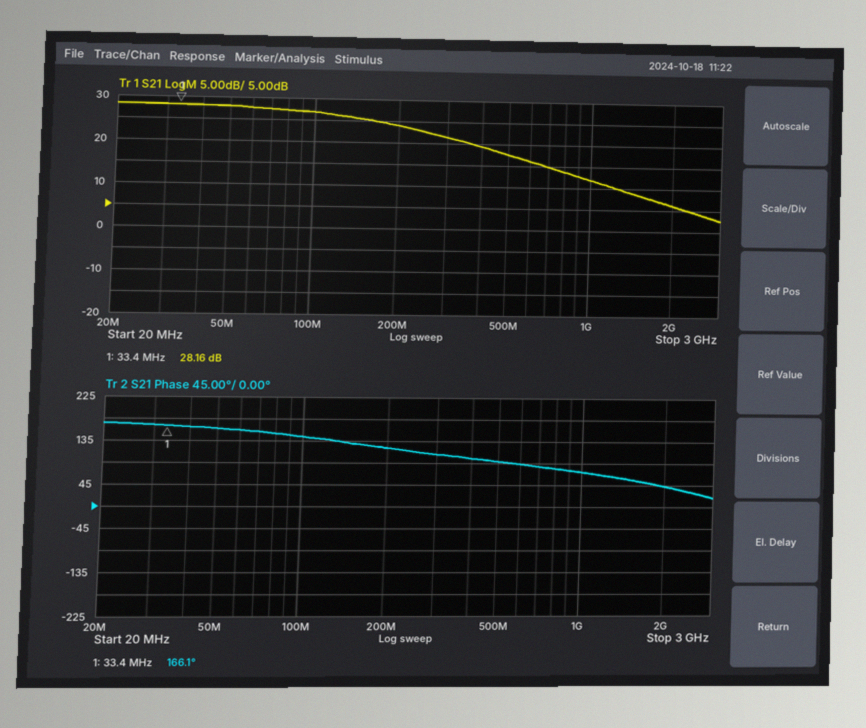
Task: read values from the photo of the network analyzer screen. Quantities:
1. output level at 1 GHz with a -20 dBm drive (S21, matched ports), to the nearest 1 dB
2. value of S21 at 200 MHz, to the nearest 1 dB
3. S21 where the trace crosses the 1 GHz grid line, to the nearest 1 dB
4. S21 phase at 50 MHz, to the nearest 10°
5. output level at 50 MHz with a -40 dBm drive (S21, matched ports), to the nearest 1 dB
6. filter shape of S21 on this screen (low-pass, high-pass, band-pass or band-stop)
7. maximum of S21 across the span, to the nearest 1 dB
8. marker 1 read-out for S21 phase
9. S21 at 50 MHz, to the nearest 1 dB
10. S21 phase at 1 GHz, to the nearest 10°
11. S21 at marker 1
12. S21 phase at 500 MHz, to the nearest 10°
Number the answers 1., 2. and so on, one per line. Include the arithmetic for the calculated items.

1. -20 dBm + (12 dB) = -8 dBm
2. 24 dB
3. 12 dB
4. 160°
5. -40 dBm + (28 dB) = -12 dBm
6. low-pass
7. 28 dB
8. 166.1°
9. 28 dB
10. 70°
11. 28.16 dB
12. 90°
